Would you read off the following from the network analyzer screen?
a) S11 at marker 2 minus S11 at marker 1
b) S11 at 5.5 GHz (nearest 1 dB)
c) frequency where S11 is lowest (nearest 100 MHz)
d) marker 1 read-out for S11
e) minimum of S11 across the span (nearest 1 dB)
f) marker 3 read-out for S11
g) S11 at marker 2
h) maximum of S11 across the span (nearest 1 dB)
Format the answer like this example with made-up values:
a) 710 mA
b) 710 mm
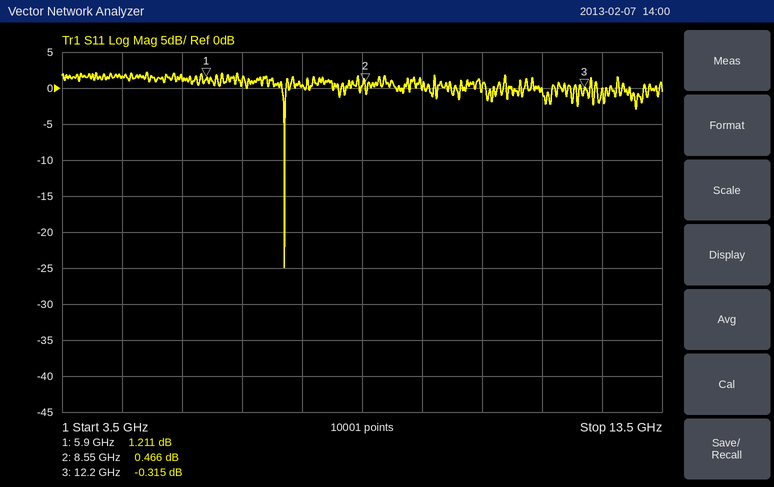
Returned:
a) -0.745 dB
b) 1 dB
c) 7.2 GHz
d) 1.211 dB
e) -25 dB
f) -0.315 dB
g) 0.466 dB
h) 2 dB
